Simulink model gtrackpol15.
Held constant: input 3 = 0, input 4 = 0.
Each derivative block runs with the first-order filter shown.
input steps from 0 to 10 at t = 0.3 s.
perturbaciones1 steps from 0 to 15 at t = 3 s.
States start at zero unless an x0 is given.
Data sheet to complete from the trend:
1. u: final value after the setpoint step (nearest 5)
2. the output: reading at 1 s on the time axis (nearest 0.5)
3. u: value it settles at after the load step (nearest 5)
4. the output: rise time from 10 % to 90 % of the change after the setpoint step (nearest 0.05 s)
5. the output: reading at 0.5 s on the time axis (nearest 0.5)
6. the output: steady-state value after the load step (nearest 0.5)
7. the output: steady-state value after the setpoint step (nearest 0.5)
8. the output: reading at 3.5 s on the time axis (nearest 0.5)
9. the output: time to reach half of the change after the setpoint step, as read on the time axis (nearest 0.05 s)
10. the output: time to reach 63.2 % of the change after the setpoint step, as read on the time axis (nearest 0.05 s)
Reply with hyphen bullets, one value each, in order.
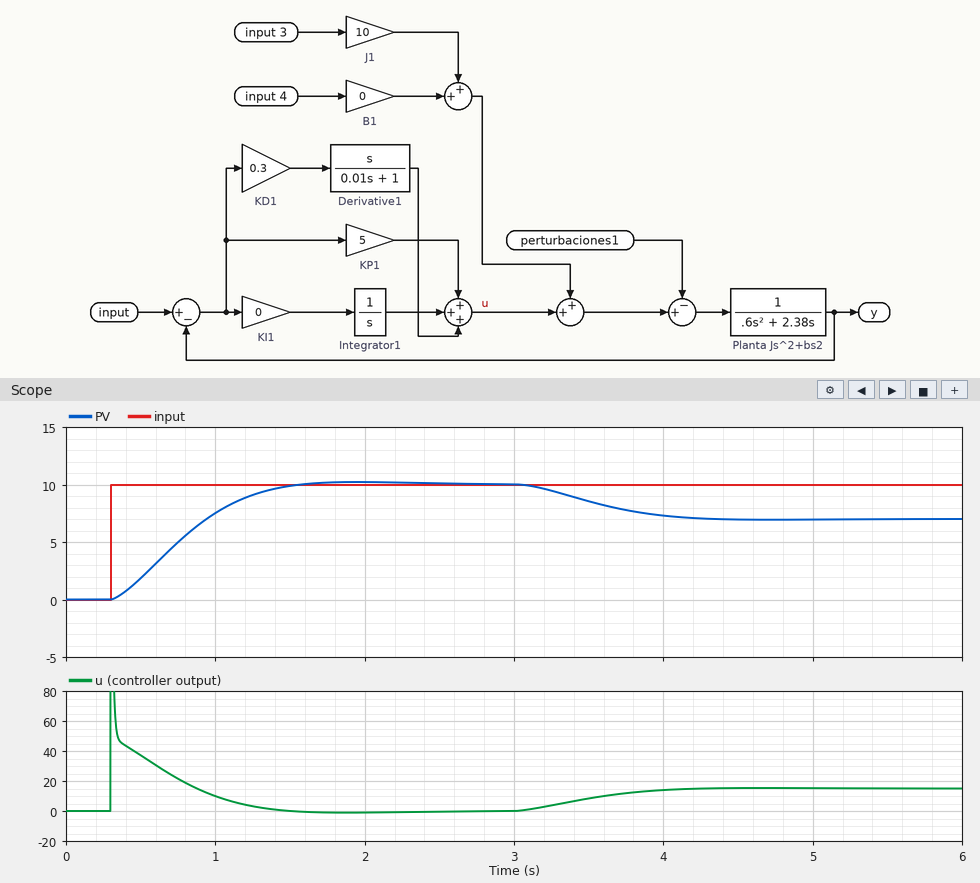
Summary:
- 0
- 7.5
- 15
- 0.80 s
- 2.0
- 7.0
- 10.0
- 8.5
- 0.75 s
- 0.85 s
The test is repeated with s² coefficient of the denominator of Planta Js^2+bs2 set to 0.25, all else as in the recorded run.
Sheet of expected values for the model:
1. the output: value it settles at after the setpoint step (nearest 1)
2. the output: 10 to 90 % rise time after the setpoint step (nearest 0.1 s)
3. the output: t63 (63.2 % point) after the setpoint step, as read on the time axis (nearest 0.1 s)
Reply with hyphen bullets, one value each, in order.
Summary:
- 10
- 1.0 s
- 0.8 s
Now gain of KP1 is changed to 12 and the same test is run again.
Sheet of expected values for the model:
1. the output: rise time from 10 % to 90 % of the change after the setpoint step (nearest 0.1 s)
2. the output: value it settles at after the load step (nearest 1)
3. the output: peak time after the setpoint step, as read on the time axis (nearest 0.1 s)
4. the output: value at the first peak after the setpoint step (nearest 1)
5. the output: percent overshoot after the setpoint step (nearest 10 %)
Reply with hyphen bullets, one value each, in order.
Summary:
- 0.4 s
- 9
- 1.1 s
- 12
- 20 %
